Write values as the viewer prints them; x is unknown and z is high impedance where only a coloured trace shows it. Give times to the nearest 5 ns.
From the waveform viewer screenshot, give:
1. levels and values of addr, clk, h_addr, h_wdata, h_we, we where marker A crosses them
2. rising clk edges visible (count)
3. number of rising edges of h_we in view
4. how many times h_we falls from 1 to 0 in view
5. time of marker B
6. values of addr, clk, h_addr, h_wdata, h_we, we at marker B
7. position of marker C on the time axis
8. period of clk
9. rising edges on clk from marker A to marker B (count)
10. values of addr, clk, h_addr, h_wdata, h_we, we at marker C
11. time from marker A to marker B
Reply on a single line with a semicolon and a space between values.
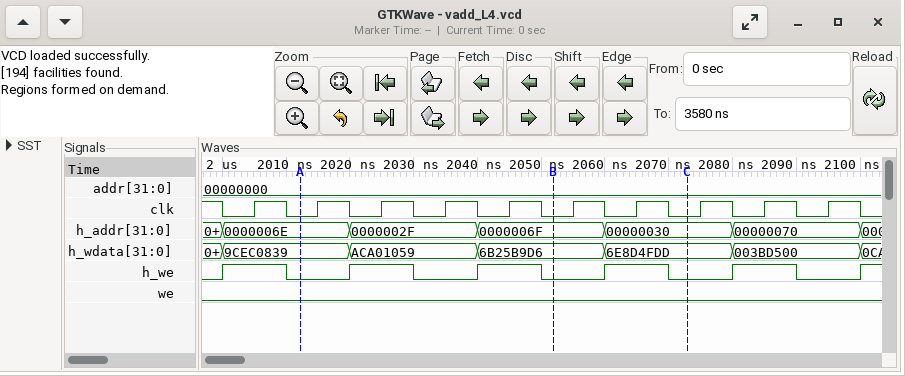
addr=00000000, clk=0, h_addr=0000006E, h_wdata=9CEC0839, h_we=0, we=0; 10; 6; 5; 2050 ns; addr=00000000, clk=0, h_addr=0000006F, h_wdata=6B25B9D6, h_we=0, we=0; 2075 ns; 10 ns; 4; addr=00000000, clk=0, h_addr=00000030, h_wdata=6E8D4FDD, h_we=0, we=0; 40 ns
